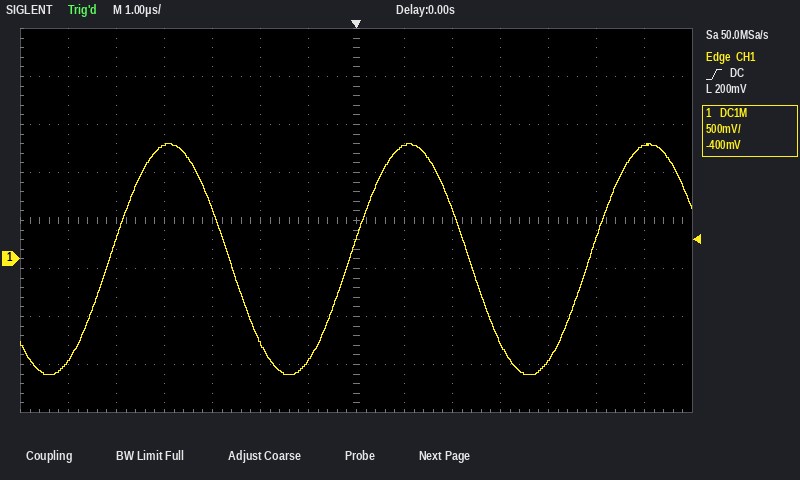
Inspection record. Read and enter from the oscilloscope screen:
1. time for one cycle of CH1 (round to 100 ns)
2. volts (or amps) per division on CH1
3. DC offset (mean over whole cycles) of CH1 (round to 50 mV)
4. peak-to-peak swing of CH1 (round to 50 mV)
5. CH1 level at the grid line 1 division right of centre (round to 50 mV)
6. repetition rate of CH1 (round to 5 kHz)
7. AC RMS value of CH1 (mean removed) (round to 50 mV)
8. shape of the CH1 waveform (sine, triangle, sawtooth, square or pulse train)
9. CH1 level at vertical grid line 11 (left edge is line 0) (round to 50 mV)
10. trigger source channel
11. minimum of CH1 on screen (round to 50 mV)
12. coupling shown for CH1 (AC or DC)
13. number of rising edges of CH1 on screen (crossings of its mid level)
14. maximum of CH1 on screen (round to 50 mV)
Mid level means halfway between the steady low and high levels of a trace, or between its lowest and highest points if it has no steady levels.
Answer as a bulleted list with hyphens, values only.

- 5.0 µs
- 500 mV
- 0 mV
- 2.40 V
- 1.20 V
- 200 kHz
- 850 mV
- sine
- -1.05 V
- CH1
- -1.20 V
- DC
- 3
- 1.20 V
